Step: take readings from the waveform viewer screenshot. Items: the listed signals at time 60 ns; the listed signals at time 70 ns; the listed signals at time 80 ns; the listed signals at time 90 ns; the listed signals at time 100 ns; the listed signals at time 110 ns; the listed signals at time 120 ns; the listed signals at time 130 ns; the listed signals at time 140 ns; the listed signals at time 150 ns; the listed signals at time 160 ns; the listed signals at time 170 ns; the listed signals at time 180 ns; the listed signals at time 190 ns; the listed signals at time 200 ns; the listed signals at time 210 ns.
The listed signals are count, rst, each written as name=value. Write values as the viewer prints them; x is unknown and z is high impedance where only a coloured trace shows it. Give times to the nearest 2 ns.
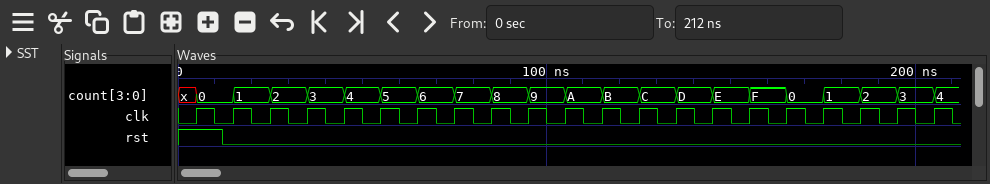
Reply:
count=5, rst=0
count=6, rst=0
count=7, rst=0
count=8, rst=0
count=9, rst=0
count=A, rst=0
count=B, rst=0
count=C, rst=0
count=D, rst=0
count=E, rst=0
count=F, rst=0
count=0, rst=0
count=1, rst=0
count=2, rst=0
count=3, rst=0
count=4, rst=0
